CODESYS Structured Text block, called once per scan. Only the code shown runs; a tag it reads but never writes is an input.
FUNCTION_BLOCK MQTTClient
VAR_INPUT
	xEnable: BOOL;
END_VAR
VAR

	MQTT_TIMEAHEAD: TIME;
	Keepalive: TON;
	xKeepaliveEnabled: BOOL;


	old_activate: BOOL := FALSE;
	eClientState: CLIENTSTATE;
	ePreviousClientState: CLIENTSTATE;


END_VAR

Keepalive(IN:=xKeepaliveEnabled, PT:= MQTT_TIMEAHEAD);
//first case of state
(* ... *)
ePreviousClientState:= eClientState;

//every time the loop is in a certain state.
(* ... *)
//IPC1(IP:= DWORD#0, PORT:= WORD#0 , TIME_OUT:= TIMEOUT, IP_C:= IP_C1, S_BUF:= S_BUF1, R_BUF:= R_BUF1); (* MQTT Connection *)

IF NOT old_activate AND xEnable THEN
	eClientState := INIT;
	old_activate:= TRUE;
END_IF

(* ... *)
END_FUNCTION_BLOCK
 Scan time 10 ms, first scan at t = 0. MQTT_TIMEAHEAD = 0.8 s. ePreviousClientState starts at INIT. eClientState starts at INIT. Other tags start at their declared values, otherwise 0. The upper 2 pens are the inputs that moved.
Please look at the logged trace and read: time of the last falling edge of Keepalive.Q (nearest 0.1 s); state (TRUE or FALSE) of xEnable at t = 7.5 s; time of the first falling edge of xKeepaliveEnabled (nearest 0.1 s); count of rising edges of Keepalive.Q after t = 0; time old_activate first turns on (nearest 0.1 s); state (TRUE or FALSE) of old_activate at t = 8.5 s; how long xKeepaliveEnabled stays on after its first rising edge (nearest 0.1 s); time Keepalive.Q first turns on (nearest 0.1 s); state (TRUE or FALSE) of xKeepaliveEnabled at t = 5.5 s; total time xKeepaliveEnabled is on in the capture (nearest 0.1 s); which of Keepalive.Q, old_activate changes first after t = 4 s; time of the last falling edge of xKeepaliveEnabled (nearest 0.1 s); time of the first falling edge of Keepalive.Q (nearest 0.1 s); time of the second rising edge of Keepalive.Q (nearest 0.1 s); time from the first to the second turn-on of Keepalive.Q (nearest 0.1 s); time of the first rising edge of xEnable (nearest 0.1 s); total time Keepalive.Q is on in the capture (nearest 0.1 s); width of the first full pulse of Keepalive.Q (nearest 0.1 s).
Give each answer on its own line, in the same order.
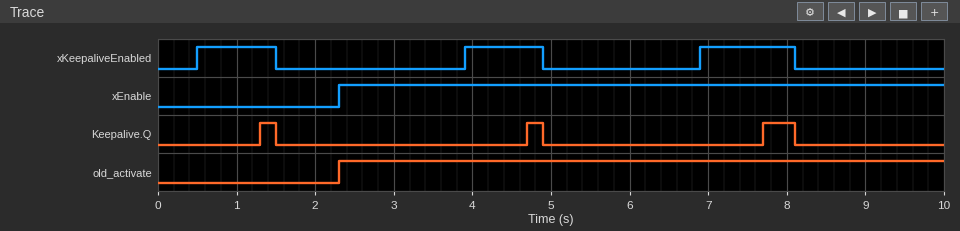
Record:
8.1 s
TRUE
1.5 s
3
2.3 s
TRUE
1.0 s
1.3 s
FALSE
3.2 s
Keepalive.Q
8.1 s
1.5 s
4.7 s
3.4 s
2.3 s
0.8 s
0.2 s
